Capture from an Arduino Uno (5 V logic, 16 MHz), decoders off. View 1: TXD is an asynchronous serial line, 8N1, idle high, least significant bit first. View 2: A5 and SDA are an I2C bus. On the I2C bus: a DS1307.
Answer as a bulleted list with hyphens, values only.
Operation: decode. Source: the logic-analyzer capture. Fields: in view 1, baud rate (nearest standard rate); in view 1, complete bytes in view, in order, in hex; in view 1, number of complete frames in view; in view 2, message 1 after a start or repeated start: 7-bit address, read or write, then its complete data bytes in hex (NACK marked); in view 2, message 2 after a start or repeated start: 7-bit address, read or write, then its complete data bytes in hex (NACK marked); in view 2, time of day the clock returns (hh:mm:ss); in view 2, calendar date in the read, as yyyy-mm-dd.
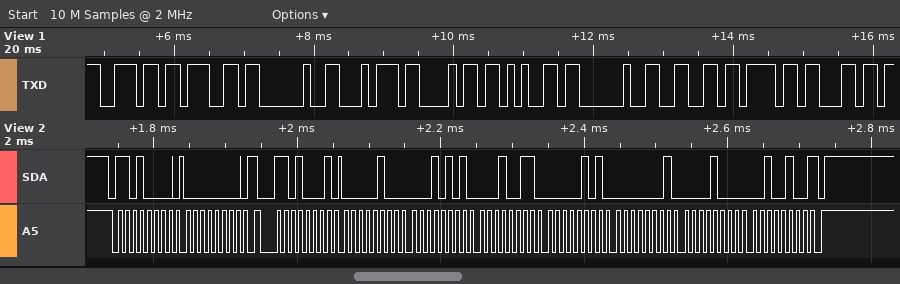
- 9600 baud
- 6E 67 20 74 68 65 20 66 6F 6C
- 10
- 0x68 write: 00
- 0x68 read: 04 15 13 05 01 08 24 NACK
- 13:15:04
- 2024-08-01
